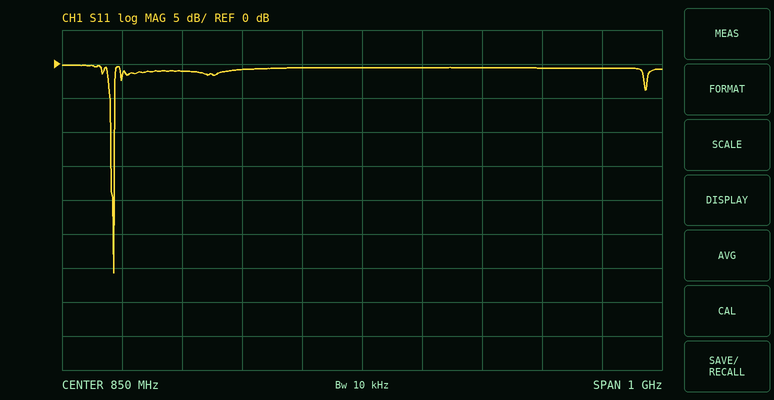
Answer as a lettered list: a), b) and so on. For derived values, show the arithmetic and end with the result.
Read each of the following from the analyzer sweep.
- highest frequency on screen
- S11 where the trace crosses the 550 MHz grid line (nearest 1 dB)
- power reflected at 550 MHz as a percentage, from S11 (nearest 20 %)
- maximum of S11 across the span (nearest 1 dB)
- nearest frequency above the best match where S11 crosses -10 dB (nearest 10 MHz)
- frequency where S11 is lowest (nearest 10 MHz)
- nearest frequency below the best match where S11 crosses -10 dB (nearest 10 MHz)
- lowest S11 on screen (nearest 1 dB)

a) 1.35 GHz
b) -1 dB
c) 10^(-1/10) ≈ 79.4 %, so 80 % to the nearest 20 %
d) 0 dB
e) 440 MHz
f) 440 MHz
g) 430 MHz
h) -31 dB
